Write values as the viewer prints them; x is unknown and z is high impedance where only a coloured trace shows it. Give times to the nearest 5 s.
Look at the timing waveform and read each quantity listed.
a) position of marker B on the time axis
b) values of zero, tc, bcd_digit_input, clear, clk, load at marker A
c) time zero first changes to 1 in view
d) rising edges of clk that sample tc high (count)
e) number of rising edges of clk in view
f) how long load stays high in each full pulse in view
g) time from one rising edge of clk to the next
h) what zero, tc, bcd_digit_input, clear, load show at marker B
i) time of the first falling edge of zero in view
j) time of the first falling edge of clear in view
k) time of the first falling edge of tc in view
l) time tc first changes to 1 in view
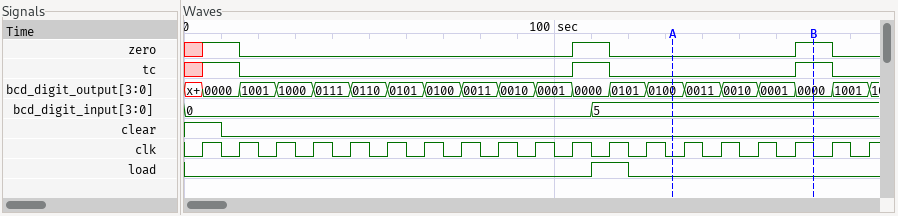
170 s
zero=0, tc=0, bcd_digit_input=5, clear=0, clk=0, load=0
5 s
3
19
10 s
10 s
zero=1, tc=1, bcd_digit_input=5, clear=0, load=0
15 s
10 s
15 s
5 s
